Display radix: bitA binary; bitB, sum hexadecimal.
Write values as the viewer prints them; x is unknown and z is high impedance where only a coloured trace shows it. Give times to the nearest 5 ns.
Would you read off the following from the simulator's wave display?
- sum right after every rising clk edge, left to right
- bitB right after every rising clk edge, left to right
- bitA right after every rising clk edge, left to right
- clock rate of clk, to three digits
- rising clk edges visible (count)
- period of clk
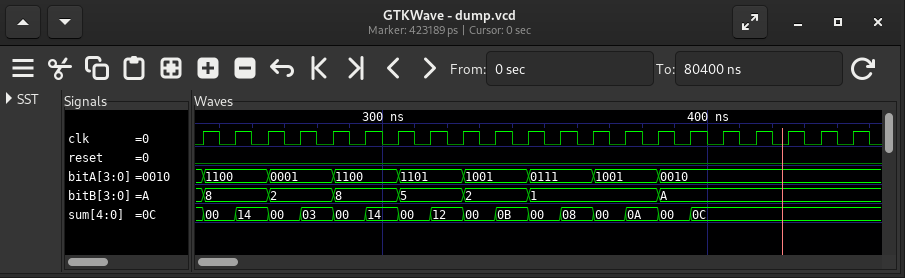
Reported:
00, 14, 00, 03, 00, 14, 00, 12, 00, 0B, 00, 08, 00, 0A, 00, 0C, 0C, 0C, 0C, 0C, 0C
8, 8, 2, 2, 8, 8, 5, 5, 2, 2, 1, 1, 1, 1, A, A, A, A, A, A, A
1100, 1100, 0001, 0001, 1100, 1100, 1101, 1101, 1001, 1001, 0111, 0111, 1001, 1001, 0010, 0010, 0010, 0010, 0010, 0010, 0010
100 MHz
21
10 ns
